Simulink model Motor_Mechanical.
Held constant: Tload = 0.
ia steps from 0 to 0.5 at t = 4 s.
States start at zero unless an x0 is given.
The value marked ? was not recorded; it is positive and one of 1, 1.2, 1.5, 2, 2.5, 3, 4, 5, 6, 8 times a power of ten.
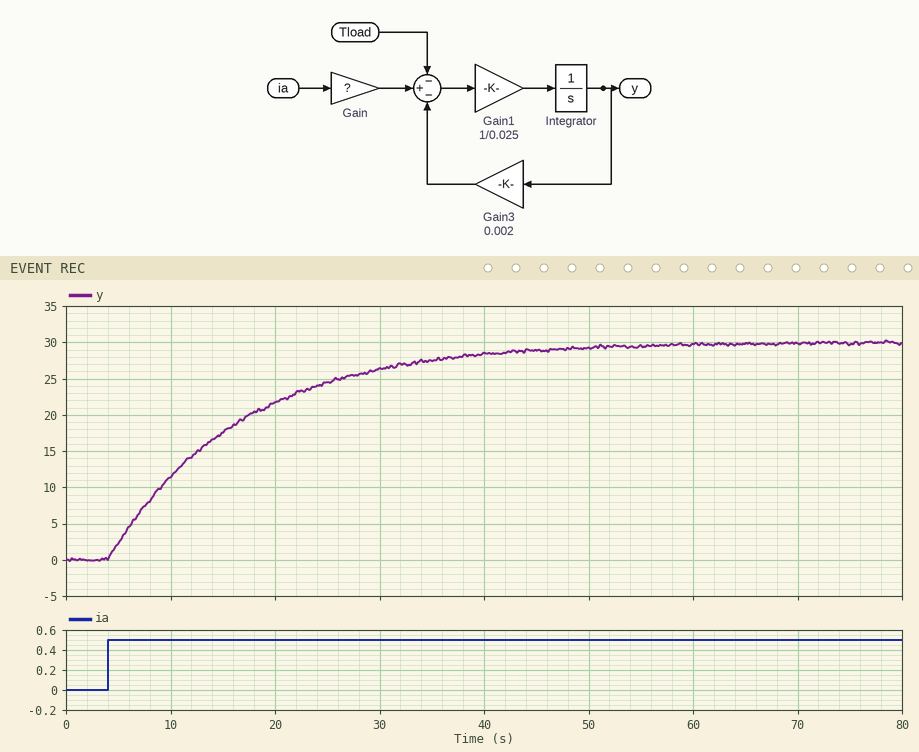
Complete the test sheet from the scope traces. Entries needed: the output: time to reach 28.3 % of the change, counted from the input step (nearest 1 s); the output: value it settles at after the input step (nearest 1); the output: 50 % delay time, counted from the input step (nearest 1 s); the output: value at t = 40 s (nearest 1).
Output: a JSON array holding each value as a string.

["4 s", "30", "9 s", "28"]
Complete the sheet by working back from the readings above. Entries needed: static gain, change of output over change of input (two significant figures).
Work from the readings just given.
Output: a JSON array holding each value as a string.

["60"]
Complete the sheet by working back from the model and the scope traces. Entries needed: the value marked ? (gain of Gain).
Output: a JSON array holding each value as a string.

["0.12"]
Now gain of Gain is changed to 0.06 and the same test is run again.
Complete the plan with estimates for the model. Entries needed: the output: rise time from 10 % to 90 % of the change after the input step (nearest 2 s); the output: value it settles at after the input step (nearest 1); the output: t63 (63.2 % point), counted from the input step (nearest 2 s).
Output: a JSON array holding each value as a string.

["28 s", "15", "12 s"]
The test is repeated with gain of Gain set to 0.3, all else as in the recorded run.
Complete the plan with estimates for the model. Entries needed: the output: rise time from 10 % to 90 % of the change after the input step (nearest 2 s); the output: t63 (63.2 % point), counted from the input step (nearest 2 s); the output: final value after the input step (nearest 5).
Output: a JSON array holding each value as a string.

["28 s", "12 s", "75"]
